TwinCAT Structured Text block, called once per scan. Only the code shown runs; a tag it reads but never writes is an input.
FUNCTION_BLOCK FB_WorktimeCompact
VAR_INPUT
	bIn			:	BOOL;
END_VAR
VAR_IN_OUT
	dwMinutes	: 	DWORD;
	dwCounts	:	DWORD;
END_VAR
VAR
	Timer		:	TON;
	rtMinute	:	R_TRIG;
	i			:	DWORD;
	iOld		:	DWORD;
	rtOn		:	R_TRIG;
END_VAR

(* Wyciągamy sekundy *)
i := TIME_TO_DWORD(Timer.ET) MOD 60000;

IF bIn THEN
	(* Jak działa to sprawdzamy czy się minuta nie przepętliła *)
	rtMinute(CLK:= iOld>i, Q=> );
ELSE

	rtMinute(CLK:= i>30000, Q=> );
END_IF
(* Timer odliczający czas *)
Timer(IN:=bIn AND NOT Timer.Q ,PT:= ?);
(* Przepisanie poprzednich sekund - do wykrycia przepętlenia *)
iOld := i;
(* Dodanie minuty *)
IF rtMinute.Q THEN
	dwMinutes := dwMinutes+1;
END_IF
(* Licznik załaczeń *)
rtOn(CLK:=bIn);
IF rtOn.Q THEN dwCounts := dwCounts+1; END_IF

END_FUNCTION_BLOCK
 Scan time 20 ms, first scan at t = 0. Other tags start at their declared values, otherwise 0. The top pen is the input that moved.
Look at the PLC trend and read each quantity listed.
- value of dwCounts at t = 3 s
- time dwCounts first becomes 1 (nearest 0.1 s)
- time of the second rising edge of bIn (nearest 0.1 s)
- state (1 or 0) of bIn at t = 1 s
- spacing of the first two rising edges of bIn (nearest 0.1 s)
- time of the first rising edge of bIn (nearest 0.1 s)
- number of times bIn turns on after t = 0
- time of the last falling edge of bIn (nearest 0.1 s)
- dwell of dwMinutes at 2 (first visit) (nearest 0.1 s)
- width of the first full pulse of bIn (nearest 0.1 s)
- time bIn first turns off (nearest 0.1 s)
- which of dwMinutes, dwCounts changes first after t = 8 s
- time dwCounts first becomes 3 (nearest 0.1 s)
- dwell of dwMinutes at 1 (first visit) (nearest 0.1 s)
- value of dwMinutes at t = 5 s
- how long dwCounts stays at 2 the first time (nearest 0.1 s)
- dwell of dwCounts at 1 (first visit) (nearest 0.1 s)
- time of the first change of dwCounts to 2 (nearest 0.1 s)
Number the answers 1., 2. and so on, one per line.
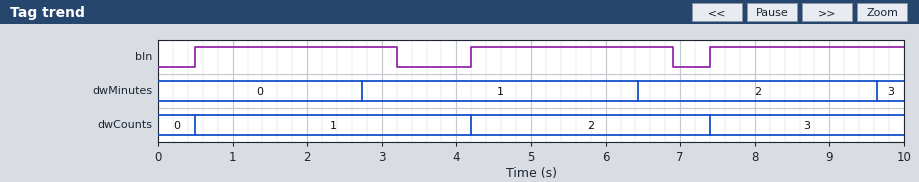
1. 1
2. 0.5 s
3. 4.2 s
4. 1
5. 3.7 s
6. 0.5 s
7. 3
8. 6.9 s
9. 3.2 s
10. 2.7 s
11. 3.2 s
12. dwMinutes
13. 7.4 s
14. 3.7 s
15. 1
16. 3.2 s
17. 3.7 s
18. 4.2 s
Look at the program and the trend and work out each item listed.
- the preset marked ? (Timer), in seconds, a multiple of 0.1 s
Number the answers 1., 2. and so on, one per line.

1. 2.2 s
